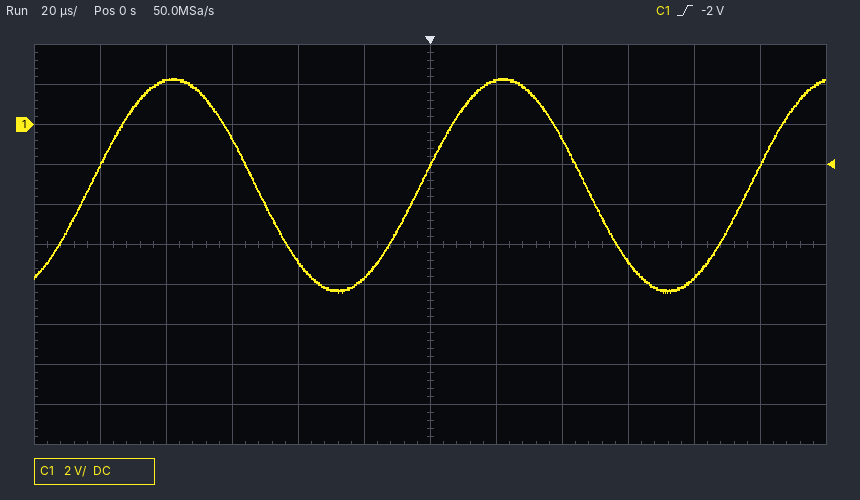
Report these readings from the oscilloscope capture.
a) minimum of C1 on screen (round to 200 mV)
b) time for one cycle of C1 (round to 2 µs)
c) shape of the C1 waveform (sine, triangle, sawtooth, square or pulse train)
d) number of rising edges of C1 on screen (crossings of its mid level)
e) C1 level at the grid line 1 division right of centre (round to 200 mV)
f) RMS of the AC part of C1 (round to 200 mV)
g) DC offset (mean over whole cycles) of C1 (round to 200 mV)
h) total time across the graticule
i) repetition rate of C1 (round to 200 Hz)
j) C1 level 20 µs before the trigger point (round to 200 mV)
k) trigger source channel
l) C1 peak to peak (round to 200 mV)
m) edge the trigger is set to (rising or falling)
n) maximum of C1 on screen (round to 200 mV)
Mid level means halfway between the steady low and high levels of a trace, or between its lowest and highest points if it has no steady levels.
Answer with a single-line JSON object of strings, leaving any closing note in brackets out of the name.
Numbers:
{"minimum of C1 on screen": "-8.4 V", "time for one cycle of C1": "100 µs", "shape of the C1 waveform": "sine", "number of rising edges of C1 on screen": "3", "C1 level at the grid line 1 division right of centre": "2.2 V", "RMS of the AC part of C1": "3.8 V", "DC offset (mean over whole cycles) of C1": "-3.0 V", "total time across the graticule": "240 µs", "repetition rate of C1": "10.0 kHz", "C1 level 20 µs before the trigger point": "-7.6 V", "trigger source channel": "C1", "C1 peak to peak": "10.8 V", "edge the trigger is set to": "rising", "maximum of C1 on screen": "2.4 V"}
